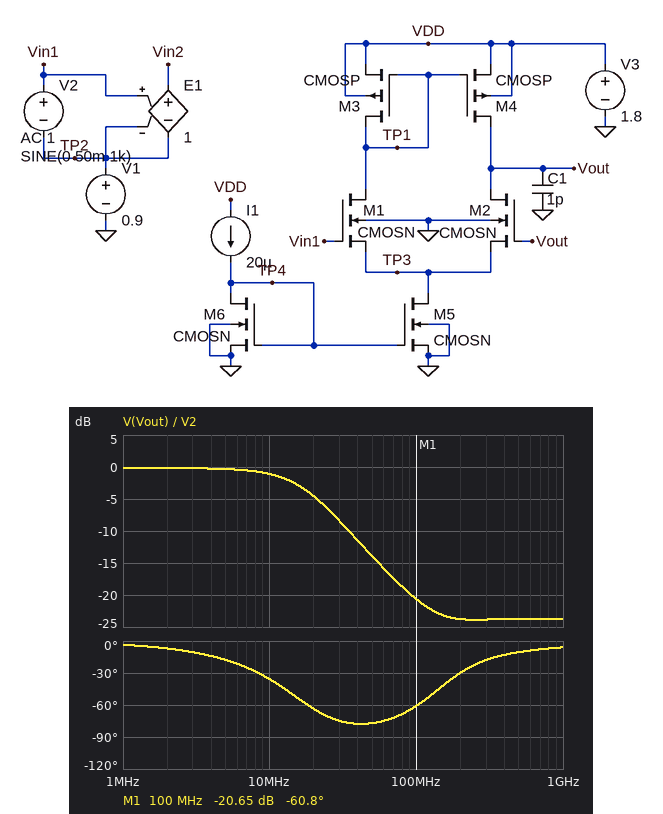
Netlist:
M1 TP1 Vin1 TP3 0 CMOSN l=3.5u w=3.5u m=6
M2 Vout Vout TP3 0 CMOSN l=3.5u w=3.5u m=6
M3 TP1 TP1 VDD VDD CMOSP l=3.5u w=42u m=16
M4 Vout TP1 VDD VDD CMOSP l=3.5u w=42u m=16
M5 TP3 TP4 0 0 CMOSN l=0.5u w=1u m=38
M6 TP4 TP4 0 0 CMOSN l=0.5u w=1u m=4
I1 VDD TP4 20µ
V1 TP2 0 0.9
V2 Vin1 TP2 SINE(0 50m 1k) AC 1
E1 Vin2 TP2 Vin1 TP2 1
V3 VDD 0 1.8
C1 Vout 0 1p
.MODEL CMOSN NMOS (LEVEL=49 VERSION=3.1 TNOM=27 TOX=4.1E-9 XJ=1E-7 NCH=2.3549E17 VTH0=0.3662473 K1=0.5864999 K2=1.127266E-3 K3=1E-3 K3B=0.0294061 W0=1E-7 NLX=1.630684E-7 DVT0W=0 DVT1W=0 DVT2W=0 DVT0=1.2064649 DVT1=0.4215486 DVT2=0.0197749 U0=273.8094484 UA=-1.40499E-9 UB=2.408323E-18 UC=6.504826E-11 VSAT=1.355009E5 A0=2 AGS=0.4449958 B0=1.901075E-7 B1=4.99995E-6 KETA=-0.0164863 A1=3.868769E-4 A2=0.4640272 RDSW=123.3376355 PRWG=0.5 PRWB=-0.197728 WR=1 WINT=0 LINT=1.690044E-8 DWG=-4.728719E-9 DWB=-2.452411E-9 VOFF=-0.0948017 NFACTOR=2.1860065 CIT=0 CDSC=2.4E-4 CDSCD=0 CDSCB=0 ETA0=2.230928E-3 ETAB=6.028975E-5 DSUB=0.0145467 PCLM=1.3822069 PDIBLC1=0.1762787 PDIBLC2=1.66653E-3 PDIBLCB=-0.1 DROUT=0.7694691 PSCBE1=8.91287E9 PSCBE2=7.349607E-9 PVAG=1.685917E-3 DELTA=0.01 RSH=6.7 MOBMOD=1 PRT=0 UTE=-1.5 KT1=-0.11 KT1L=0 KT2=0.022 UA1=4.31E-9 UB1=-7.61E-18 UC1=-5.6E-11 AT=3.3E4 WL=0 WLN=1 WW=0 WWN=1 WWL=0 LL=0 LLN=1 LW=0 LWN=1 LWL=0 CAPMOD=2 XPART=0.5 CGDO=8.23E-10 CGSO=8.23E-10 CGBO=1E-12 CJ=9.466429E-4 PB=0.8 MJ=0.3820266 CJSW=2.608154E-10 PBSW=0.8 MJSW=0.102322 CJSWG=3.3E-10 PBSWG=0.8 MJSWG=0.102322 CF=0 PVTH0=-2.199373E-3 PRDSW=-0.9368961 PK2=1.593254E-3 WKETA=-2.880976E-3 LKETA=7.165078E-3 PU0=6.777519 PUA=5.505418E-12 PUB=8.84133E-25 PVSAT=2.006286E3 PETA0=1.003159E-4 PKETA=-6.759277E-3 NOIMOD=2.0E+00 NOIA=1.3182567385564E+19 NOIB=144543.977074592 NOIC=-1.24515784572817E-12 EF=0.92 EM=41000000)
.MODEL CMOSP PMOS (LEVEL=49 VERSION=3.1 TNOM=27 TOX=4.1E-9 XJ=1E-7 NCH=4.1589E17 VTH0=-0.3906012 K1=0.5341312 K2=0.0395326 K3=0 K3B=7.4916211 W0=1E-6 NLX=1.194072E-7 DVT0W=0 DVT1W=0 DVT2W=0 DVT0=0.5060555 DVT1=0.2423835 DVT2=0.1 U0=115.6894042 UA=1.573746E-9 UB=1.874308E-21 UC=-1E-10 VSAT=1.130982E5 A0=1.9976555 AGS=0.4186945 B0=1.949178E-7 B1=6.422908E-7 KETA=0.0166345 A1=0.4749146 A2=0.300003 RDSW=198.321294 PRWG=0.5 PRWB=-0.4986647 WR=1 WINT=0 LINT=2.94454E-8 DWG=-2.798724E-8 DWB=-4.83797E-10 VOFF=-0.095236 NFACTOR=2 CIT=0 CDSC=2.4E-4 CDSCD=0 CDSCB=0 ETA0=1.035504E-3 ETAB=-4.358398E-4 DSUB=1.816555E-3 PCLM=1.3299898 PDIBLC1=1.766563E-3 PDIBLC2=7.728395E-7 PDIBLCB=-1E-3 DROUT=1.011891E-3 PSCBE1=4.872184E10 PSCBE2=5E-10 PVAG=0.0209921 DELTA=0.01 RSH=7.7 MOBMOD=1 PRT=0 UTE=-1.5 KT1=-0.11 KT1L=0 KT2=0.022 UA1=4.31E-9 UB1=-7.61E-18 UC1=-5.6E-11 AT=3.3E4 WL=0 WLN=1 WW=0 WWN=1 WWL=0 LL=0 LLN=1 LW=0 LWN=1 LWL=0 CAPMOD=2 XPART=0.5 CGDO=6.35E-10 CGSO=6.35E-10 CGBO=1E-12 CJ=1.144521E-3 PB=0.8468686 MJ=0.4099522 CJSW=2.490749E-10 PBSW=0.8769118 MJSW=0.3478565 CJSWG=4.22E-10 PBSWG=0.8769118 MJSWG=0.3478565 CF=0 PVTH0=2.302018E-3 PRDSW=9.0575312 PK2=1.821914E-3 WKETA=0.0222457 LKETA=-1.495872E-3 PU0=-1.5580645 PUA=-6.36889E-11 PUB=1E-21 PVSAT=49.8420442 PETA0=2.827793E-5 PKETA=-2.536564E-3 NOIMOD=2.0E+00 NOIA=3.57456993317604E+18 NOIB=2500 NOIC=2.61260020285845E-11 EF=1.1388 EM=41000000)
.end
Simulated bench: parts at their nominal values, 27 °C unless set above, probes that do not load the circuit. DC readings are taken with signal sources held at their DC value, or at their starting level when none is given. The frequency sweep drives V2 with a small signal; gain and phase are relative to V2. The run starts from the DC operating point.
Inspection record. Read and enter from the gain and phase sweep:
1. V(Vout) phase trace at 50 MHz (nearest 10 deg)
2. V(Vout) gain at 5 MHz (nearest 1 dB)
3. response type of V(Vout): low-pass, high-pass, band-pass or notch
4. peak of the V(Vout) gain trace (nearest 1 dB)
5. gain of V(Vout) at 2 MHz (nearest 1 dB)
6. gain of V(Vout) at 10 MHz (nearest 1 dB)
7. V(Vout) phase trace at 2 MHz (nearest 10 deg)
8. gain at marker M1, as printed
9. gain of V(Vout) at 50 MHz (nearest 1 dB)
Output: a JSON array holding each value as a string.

["-80 deg", "0 dB", "low-pass", "0 dB", "0 dB", "-1 dB", "-10 deg", "-20.65 dB", "-14 dB"]
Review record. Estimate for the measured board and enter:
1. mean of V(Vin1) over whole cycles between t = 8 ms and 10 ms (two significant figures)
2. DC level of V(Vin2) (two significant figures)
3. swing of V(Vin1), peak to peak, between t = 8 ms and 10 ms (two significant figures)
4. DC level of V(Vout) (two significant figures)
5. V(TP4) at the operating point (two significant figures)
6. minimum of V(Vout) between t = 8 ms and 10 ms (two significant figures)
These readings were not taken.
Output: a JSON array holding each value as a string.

["900 mV", "900 mV", "100 mV", "910 mV", "570 mV", "860 mV"]
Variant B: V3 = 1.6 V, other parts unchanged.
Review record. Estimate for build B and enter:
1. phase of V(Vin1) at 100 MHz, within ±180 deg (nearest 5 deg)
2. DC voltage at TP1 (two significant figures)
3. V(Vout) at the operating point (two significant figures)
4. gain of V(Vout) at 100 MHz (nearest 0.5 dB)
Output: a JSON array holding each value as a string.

["0 deg", "1.1 V", "900 mV", "-21.0 dB"]
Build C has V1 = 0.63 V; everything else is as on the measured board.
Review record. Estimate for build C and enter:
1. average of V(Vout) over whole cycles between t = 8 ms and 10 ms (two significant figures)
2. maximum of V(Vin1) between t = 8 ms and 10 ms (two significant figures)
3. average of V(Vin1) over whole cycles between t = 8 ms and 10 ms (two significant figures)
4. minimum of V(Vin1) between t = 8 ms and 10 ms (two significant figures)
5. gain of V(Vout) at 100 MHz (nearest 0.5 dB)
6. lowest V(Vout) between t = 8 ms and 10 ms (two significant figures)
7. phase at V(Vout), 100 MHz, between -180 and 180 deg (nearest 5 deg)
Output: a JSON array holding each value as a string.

["640 mV", "680 mV", "630 mV", "580 mV", "-26.5 dB", "590 mV", "45 deg"]
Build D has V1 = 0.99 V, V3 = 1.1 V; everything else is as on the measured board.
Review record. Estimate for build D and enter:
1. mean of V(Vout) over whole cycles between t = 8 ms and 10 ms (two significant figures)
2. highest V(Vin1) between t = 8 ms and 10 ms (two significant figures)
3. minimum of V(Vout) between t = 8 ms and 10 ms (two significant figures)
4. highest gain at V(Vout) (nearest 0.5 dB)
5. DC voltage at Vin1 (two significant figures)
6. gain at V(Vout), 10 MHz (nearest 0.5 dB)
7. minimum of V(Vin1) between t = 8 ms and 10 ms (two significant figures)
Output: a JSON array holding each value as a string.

["970 mV", "1.0 V", "930 mV", "-2.0 dB", "990 mV", "-3.5 dB", "940 mV"]
